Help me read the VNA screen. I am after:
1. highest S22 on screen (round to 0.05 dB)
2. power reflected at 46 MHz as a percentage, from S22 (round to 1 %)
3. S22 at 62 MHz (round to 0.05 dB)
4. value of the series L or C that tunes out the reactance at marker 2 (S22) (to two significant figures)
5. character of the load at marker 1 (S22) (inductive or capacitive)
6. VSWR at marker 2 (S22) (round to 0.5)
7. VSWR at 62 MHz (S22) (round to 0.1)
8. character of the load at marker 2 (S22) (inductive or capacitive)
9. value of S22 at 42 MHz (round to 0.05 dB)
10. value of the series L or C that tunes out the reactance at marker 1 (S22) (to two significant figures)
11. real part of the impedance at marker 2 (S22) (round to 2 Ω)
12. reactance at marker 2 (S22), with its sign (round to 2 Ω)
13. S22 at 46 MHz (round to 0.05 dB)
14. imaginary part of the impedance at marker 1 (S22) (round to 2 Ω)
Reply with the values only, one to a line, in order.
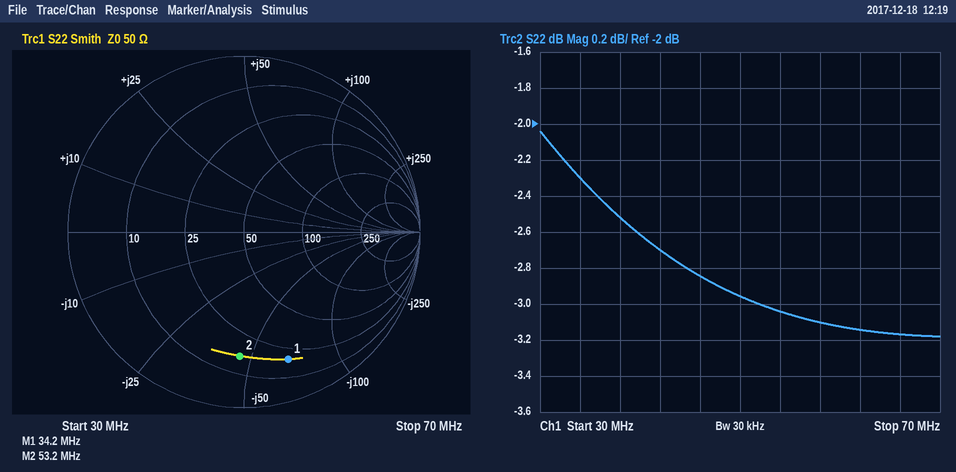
-2.05 dB
52 %
-3.15 dB
140 nH
capacitive
6.0
5.6
capacitive
-2.70 dB
310 nH
16 Ω
-46 Ω
-2.85 dB
-66 Ω
